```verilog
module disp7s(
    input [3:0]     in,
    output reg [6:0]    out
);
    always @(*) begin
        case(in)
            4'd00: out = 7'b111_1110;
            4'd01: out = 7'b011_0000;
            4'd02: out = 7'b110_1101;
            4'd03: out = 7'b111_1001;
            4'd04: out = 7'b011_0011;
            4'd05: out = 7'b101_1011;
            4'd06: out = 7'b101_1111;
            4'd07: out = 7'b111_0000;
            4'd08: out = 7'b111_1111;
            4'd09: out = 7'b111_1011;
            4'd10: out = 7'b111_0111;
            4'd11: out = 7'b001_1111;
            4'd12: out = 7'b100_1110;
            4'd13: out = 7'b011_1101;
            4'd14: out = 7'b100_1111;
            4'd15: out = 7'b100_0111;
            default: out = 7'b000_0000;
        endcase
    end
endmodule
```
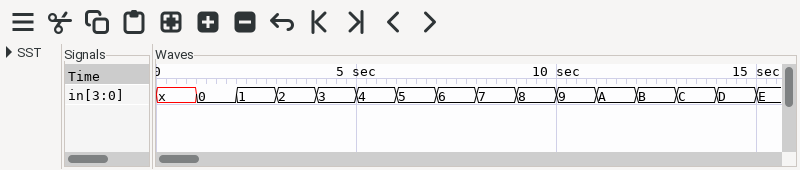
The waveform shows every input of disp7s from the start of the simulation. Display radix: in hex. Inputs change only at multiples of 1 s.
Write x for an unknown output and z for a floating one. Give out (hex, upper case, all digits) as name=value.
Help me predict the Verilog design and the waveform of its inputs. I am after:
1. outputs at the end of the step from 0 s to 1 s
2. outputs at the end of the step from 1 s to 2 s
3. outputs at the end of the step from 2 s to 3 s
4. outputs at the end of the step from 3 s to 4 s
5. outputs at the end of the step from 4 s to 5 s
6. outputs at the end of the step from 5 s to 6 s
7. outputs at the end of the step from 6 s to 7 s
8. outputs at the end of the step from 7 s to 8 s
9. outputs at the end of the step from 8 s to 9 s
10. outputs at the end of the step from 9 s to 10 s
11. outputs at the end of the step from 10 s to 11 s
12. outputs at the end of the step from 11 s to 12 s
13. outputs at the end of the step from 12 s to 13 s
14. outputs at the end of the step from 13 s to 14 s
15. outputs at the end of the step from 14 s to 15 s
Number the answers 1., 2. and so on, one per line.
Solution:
1. out=x
2. out=7E
3. out=30
4. out=6D
5. out=79
6. out=33
7. out=5B
8. out=5F
9. out=70
10. out=7F
11. out=7B
12. out=77
13. out=1F
14. out=4E
15. out=3D
